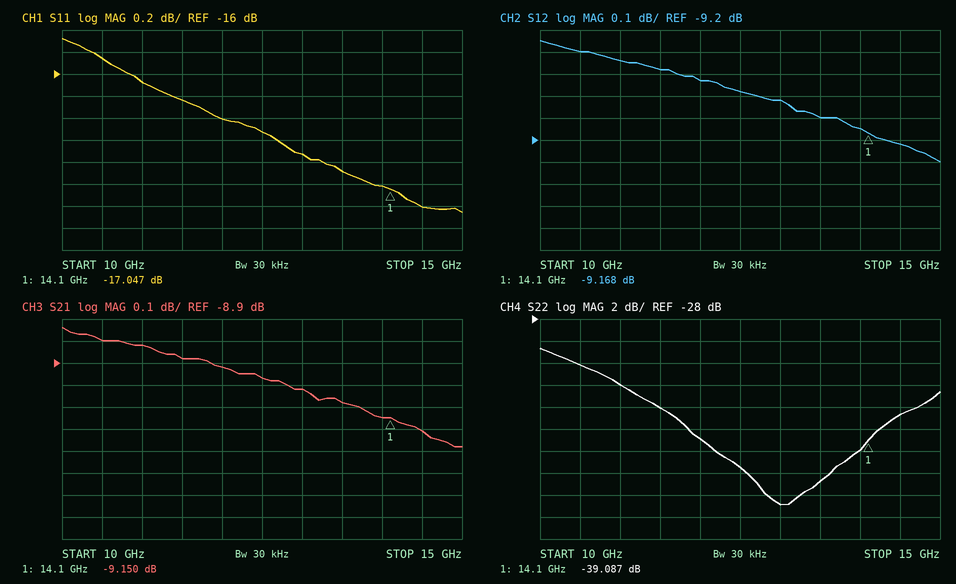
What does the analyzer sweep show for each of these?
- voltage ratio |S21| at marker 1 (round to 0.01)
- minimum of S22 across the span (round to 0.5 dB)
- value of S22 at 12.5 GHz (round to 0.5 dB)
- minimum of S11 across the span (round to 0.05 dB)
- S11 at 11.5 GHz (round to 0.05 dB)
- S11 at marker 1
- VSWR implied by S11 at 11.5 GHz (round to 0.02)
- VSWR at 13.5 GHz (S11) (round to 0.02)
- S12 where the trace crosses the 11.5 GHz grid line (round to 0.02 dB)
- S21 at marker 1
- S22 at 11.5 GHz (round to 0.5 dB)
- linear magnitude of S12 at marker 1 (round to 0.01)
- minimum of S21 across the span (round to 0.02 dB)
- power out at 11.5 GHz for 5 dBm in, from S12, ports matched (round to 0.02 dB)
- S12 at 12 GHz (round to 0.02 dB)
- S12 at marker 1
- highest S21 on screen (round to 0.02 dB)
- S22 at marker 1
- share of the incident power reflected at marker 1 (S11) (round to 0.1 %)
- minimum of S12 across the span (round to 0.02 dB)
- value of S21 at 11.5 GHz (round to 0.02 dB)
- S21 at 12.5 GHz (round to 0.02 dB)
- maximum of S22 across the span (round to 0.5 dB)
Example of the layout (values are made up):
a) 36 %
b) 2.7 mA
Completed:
a) 0.35
b) -45.0 dB
c) -41.5 dB
d) -17.25 dB
e) -16.25 dB
f) -17.047 dB
g) 1.36
h) 1.34
i) -8.88 dB
j) -9.150 dB
k) -36.0 dB
l) 0.35
m) -9.28 dB
n) -3.88 dBm
o) -8.92 dB
p) -9.168 dB
q) -8.74 dB
r) -39.087 dB
s) 2.0 %
t) -9.30 dB
u) -8.88 dB
v) -8.96 dB
w) -30.5 dB
